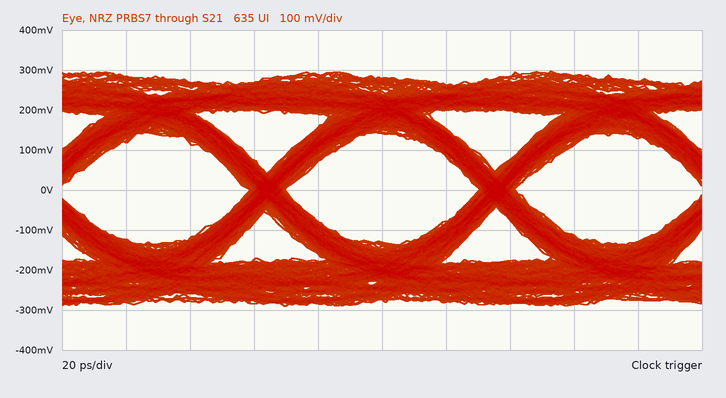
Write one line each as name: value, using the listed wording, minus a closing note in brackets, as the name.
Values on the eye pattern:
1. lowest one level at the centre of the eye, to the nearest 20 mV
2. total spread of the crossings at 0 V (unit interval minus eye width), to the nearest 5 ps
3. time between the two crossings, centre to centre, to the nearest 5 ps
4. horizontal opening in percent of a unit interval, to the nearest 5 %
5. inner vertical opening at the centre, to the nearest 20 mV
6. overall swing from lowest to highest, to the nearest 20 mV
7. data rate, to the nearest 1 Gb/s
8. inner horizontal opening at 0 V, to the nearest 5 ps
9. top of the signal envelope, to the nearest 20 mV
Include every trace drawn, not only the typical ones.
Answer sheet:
lowest one level at the centre of the eye, to the nearest 20 mV: 140 mV
total spread of the crossings at 0 V (unit interval minus eye width), to the nearest 5 ps: 10 ps
time between the two crossings, centre to centre, to the nearest 5 ps: 70 ps
horizontal opening in percent of a unit interval, to the nearest 5 %: 85 %
inner vertical opening at the centre, to the nearest 20 mV: 280 mV
overall swing from lowest to highest, to the nearest 20 mV: 580 mV
data rate, to the nearest 1 Gb/s: 14 Gb/s
inner horizontal opening at 0 V, to the nearest 5 ps: 60 ps
top of the signal envelope, to the nearest 20 mV: 300 mV
